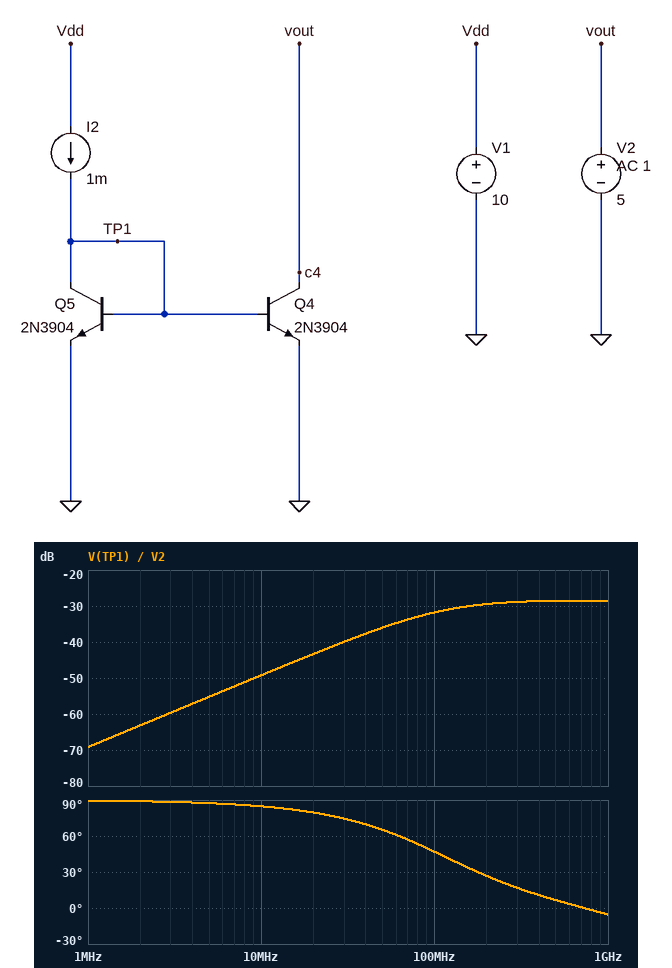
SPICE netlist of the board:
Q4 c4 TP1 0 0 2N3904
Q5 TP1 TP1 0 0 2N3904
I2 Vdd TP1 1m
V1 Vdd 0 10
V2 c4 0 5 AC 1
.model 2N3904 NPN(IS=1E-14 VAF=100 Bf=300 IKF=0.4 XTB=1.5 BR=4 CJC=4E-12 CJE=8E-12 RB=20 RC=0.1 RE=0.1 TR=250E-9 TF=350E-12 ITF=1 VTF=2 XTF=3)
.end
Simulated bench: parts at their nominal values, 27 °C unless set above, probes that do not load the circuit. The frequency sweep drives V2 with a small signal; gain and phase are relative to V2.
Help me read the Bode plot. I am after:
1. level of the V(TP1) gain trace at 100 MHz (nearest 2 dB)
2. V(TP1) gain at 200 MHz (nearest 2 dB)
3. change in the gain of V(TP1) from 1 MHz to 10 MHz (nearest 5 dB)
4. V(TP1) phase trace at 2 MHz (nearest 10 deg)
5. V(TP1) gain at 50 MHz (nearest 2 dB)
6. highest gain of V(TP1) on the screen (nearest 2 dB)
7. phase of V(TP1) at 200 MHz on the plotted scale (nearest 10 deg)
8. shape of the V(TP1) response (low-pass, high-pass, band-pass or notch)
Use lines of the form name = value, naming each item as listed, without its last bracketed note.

level of the V(TP1) gain trace at 100 MHz = -32 dB
V(TP1) gain at 200 MHz = -30 dB
change in the gain of V(TP1) from 1 MHz to 10 MHz = 20 dB
V(TP1) phase trace at 2 MHz = 90 deg
V(TP1) gain at 50 MHz = -36 dB
highest gain of V(TP1) on the screen = -28 dB
phase of V(TP1) at 200 MHz on the plotted scale = 30 deg
shape of the V(TP1) response = high-pass
